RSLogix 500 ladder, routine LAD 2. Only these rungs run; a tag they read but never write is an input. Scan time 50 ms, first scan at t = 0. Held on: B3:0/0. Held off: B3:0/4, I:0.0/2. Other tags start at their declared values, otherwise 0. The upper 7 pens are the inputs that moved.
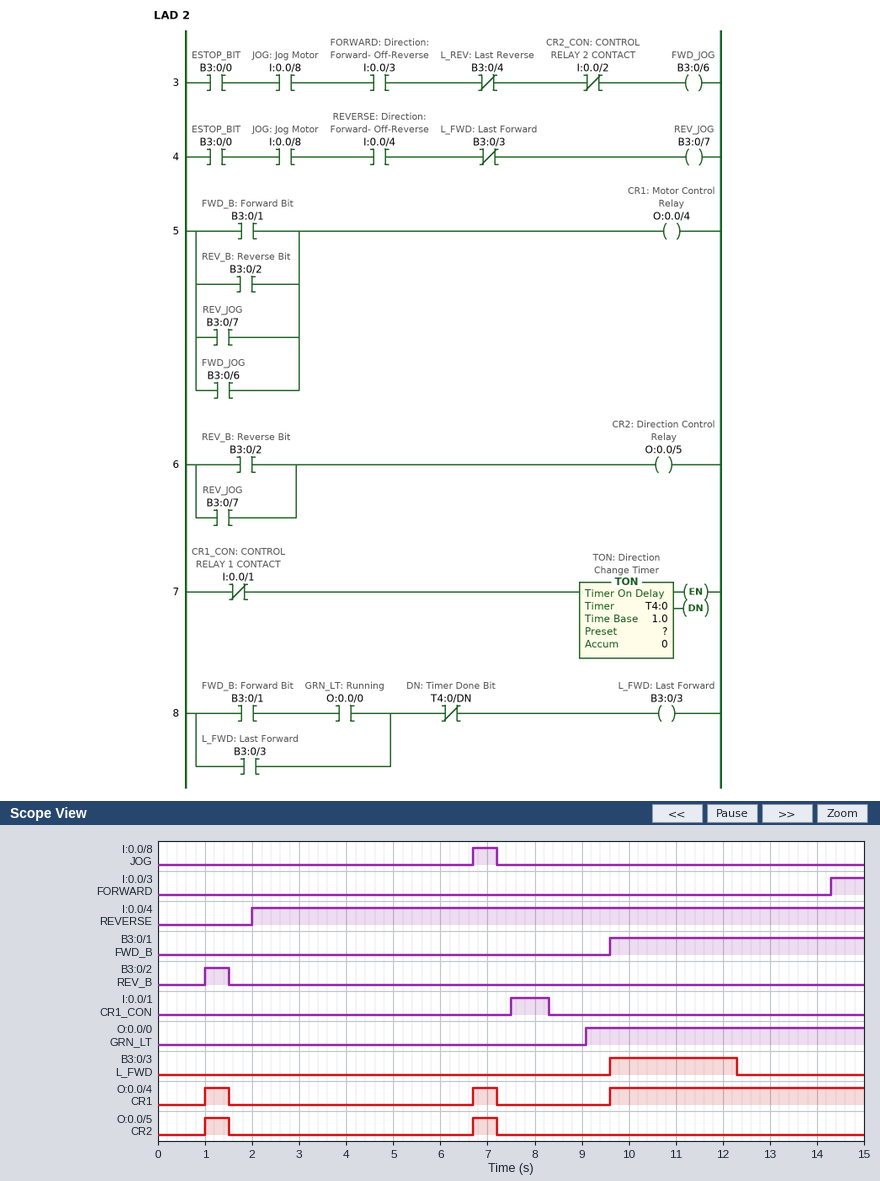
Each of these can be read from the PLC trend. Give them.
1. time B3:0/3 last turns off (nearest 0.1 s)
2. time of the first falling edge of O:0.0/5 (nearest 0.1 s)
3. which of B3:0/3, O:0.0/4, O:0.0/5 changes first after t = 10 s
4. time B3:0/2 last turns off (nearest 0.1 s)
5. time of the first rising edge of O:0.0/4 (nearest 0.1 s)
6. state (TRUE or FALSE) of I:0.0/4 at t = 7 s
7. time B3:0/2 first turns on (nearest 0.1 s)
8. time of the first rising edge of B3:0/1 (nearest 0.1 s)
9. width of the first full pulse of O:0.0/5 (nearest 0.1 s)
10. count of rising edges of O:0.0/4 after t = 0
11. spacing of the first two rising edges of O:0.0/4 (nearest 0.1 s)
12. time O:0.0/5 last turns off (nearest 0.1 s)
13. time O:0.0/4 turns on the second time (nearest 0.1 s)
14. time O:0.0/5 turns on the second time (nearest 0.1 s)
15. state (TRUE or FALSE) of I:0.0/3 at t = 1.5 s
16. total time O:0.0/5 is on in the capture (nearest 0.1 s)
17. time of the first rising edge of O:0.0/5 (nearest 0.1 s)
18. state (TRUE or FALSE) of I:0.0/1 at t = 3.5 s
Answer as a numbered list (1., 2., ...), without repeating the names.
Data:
1. 12.3 s
2. 1.5 s
3. B3:0/3
4. 1.5 s
5. 1.0 s
6. TRUE
7. 1.0 s
8. 9.6 s
9. 0.5 s
10. 3
11. 5.7 s
12. 7.2 s
13. 6.7 s
14. 6.7 s
15. FALSE
16. 1.0 s
17. 1.0 s
18. FALSE
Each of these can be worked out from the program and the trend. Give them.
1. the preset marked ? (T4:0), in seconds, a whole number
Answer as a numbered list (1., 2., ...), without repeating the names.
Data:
1. 4 s
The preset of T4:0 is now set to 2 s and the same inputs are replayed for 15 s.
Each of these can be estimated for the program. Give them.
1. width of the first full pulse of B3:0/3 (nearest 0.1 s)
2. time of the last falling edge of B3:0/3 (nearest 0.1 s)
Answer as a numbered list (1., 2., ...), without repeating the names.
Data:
1. 0.7 s
2. 10.3 s
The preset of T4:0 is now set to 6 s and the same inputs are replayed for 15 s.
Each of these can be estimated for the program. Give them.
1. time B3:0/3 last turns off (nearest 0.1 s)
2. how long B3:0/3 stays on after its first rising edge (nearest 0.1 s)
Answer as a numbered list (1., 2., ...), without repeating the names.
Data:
1. 14.3 s
2. 4.7 s
